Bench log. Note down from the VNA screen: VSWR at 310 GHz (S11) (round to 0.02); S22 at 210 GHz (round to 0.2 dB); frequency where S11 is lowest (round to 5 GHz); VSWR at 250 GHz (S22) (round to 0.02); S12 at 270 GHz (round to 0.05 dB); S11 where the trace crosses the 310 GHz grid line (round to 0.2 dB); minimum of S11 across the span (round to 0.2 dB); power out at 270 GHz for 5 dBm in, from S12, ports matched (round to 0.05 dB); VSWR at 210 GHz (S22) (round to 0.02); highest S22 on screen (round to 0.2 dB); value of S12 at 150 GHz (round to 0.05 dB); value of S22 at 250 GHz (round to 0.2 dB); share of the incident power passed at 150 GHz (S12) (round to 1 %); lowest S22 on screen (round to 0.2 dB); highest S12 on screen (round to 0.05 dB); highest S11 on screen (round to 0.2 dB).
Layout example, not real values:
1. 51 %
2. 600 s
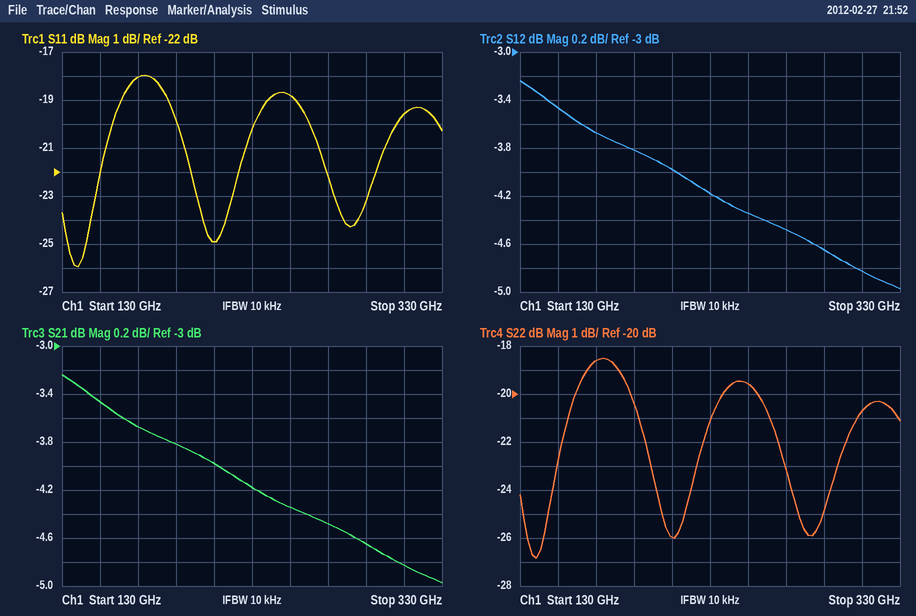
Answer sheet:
1. 1.24
2. -26.0 dB
3. 140 GHz
4. 1.24
5. -4.50 dB
6. -19.6 dB
7. -26.0 dB
8. 0.50 dBm
9. 1.10
10. -18.6 dB
11. -3.45 dB
12. -19.6 dB
13. 45 %
14. -26.8 dB
15. -3.25 dB
16. -18.0 dB
